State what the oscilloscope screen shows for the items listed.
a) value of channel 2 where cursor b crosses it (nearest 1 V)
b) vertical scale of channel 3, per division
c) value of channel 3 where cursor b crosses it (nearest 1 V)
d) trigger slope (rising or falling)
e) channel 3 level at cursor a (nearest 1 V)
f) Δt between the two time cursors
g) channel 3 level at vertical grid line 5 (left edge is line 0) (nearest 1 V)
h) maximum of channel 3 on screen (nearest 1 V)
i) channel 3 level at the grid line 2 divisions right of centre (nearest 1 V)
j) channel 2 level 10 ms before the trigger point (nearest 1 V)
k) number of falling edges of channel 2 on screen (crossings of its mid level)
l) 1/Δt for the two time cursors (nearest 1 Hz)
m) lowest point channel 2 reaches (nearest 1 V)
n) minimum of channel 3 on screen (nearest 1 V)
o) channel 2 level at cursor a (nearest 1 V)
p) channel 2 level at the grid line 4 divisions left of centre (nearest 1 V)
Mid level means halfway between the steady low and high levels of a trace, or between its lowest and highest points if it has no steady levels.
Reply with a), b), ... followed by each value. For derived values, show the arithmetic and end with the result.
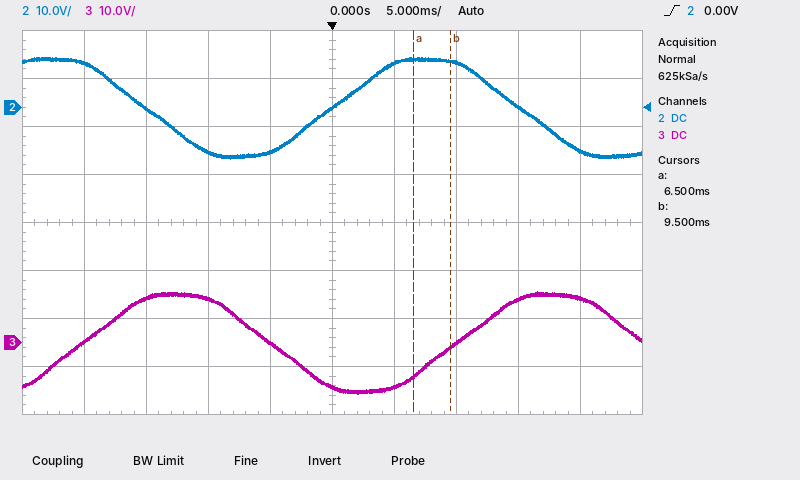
a) 10 V
b) 10 V
c) -1 V
d) rising
e) -7 V
f) 9.5 ms − (6.5 ms) = 3.0 ms
g) -9 V
h) 11 V
i) 0 V
j) -9 V
k) 2
l) 1 / 3.0 ms ≈ 333 Hz
m) -11 V
n) -11 V
o) 10 V
p) 9 V
